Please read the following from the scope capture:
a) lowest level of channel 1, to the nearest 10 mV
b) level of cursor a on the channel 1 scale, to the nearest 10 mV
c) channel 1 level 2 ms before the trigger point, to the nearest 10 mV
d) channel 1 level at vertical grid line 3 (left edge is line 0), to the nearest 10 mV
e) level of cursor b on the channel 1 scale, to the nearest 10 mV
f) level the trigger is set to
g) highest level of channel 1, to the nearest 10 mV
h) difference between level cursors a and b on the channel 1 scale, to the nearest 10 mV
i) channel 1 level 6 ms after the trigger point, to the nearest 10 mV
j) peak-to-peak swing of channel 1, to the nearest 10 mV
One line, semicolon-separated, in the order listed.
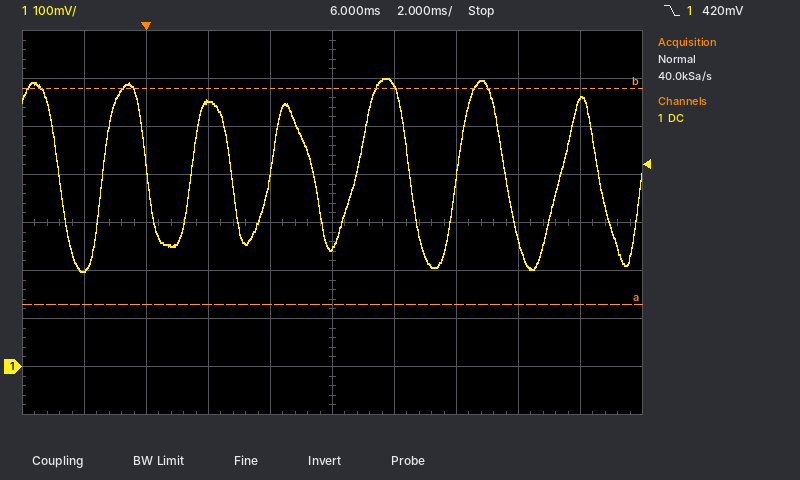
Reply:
200 mV; 130 mV; 200 mV; 550 mV; 580 mV; 420 mV; 600 mV; 450 mV; 250 mV; 400 mV
